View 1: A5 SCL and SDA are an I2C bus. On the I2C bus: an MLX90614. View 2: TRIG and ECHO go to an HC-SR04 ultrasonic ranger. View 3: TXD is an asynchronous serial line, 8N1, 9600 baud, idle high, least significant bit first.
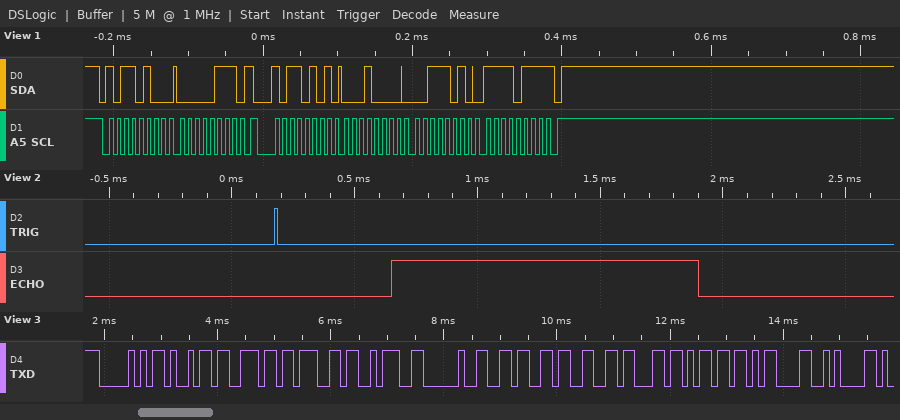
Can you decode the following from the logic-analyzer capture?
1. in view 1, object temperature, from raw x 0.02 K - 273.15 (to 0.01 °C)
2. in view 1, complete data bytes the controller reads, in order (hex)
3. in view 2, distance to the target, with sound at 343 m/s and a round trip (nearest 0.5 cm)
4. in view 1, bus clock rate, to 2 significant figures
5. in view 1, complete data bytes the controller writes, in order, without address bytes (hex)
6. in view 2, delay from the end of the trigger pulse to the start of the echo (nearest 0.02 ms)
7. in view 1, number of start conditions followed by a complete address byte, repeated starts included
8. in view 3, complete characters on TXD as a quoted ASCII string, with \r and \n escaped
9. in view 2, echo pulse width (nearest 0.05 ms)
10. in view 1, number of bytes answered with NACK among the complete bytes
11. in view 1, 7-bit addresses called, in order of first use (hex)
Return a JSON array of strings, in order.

["24.13 °C", "10 3A F7", "21.5 cm", "100 kHz", "07", "0.46 ms", "2", "\"Ping: 63cm\\r\\n\"", "1.25 ms", "1", "0x5A"]
